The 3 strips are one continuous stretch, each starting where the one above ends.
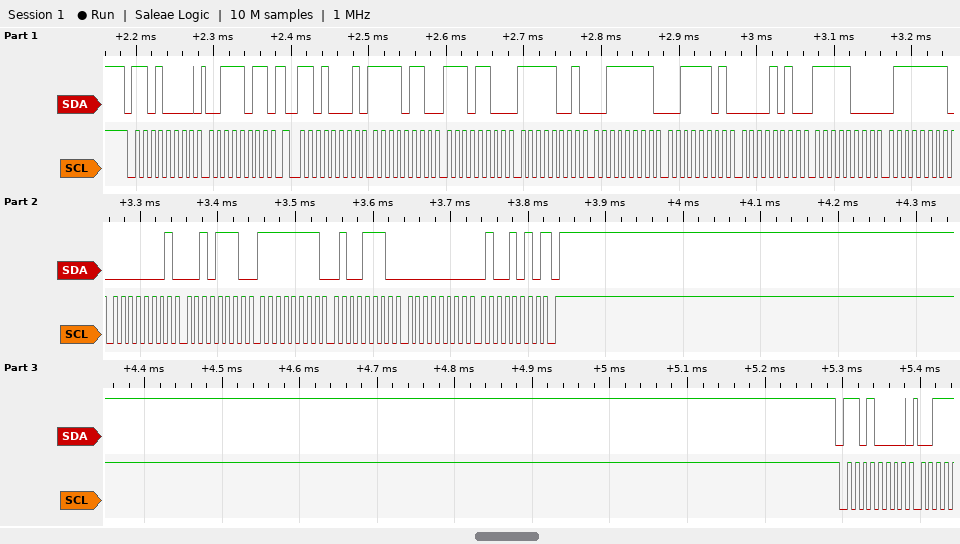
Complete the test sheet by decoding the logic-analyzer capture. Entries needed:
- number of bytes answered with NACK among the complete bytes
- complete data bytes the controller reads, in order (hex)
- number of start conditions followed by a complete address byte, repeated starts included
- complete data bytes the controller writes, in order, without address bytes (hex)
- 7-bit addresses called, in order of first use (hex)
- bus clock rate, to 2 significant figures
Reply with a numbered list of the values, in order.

1. 1
2. F6 EC F9 3F 3D 0A F8 7F 01 2E FF 4E 00 4A
3. 3
4. 3B
5. 0x68
6. 100 kHz
